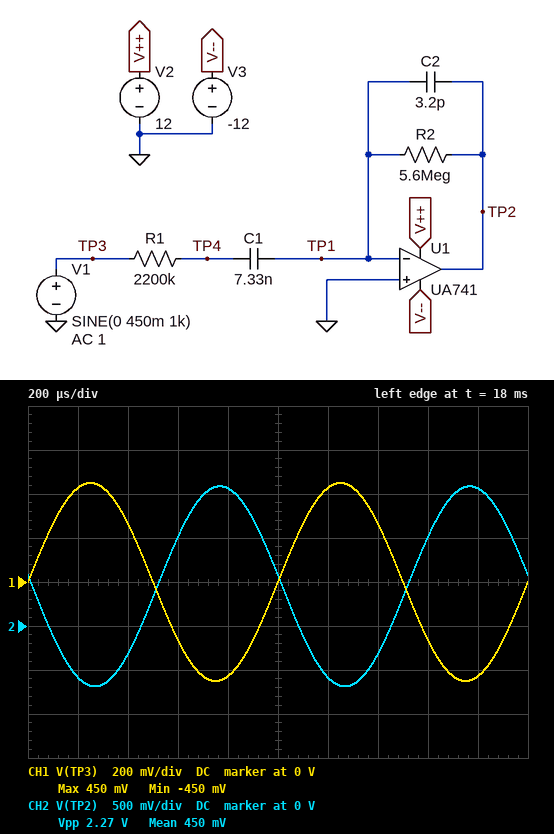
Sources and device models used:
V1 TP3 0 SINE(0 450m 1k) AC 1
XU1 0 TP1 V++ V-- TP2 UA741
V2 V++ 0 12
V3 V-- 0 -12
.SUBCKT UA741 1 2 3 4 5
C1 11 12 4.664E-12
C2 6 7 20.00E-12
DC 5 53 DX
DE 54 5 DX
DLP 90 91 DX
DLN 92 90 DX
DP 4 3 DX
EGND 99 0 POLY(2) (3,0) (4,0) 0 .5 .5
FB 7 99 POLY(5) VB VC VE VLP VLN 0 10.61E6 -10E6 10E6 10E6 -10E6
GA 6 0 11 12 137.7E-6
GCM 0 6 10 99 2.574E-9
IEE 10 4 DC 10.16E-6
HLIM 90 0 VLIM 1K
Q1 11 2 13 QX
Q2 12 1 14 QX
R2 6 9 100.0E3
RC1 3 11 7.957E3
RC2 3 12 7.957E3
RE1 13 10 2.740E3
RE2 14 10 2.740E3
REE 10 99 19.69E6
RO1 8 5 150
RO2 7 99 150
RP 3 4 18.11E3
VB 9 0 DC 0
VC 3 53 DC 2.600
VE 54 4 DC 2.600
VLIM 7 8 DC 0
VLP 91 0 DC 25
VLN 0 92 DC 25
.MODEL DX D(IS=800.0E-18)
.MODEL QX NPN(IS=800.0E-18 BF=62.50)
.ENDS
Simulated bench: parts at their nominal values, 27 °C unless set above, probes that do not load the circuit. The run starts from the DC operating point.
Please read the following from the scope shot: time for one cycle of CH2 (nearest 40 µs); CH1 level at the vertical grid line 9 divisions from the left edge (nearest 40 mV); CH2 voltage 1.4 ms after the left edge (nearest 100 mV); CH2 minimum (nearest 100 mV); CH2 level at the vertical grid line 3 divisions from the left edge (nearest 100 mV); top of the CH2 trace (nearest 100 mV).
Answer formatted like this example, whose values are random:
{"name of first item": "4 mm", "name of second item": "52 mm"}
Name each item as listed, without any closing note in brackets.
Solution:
{"time for one cycle of CH2": "1.00 ms", "CH1 level at the vertical grid line 9 divisions from the left edge": "-440 mV", "CH2 voltage 1.4 ms after the left edge": "-300 mV", "CH2 minimum": "-700 mV", "CH2 level at the vertical grid line 3 divisions from the left edge": "1.0 V", "top of the CH2 trace": "1.6 V"}
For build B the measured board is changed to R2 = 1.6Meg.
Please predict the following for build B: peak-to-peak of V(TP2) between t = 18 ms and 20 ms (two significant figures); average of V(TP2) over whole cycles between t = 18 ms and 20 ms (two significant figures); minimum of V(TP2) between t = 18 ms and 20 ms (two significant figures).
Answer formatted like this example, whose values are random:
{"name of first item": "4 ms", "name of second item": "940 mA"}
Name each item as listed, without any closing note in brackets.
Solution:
{"peak-to-peak of V(TP2) between t = 18 ms and 20 ms": "650 mV", "average of V(TP2) over whole cycles between t = 18 ms and 20 ms": "130 mV", "minimum of V(TP2) between t = 18 ms and 20 ms": "-200 mV"}
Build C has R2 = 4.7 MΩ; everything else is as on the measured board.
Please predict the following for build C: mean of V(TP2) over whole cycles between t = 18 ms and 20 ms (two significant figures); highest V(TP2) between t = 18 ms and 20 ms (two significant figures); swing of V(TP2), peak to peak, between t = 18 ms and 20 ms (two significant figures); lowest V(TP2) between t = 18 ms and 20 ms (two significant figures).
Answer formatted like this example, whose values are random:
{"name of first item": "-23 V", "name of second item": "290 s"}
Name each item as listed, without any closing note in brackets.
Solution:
{"mean of V(TP2) over whole cycles between t = 18 ms and 20 ms": "380 mV", "highest V(TP2) between t = 18 ms and 20 ms": "1.3 V", "swing of V(TP2), peak to peak, between t = 18 ms and 20 ms": "1.9 V", "lowest V(TP2) between t = 18 ms and 20 ms": "-580 mV"}
